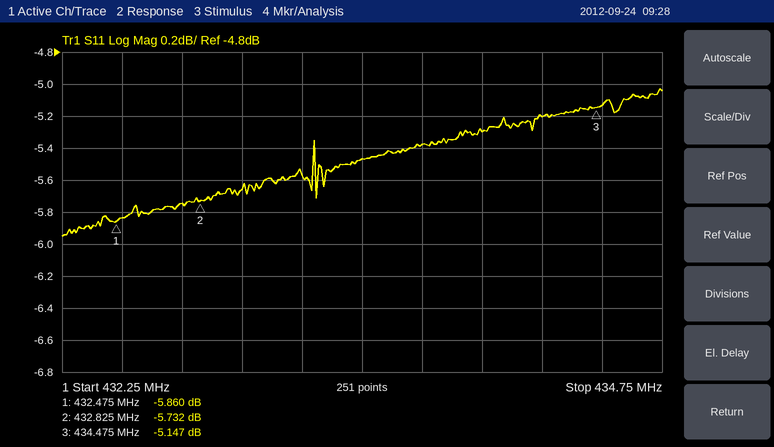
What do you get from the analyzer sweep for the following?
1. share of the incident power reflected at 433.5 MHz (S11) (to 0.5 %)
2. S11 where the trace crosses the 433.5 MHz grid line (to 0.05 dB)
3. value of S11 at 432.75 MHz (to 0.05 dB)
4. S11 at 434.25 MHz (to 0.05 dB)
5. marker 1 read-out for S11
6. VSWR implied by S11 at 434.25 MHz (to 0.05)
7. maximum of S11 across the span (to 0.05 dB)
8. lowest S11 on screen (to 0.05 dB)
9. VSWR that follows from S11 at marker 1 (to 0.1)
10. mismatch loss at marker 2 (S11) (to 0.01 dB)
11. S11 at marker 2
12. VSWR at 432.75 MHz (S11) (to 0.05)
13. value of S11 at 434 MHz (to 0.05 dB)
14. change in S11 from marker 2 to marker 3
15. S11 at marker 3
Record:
28.5 %
-5.45 dB
-5.75 dB
-5.20 dB
-5.860 dB
3.45
-5.05 dB
-5.95 dB
3.1
1.35 dB
-5.732 dB
3.15
-5.30 dB
0.585 dB
-5.147 dB
